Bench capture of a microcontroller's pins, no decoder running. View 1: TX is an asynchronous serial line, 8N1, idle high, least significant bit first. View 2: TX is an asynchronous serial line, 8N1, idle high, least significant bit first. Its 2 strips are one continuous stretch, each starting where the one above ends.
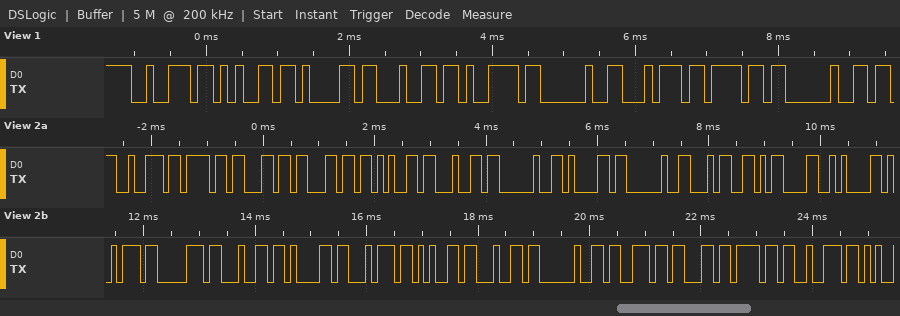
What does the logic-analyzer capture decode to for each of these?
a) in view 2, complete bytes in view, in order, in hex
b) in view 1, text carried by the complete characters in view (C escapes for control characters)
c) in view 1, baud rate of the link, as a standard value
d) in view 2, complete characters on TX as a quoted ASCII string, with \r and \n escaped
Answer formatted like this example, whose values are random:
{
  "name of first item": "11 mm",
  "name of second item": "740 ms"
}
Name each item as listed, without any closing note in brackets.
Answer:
{
  "in view 2, complete bytes in view, in order, in hex": "0x72 0x6F 0x6C 0x6C 0x65 0x64 0x20 0x61 0x20 0x34 0x0D 0x0A 0x75 0x70 0x64 0x61 0x74 0x65 0x64 0x20 0x73 0x63 0x6F 0x72",
  "in view 1, text carried by the complete characters in view": "\"ready to \"",
  "in view 1, baud rate of the link, as a standard value": "9600 baud",
  "in view 2, complete characters on TX as a quoted ASCII string, with \\r and \\n escaped": "\"rolled a 4\\r\\nupdated scor\""
}
